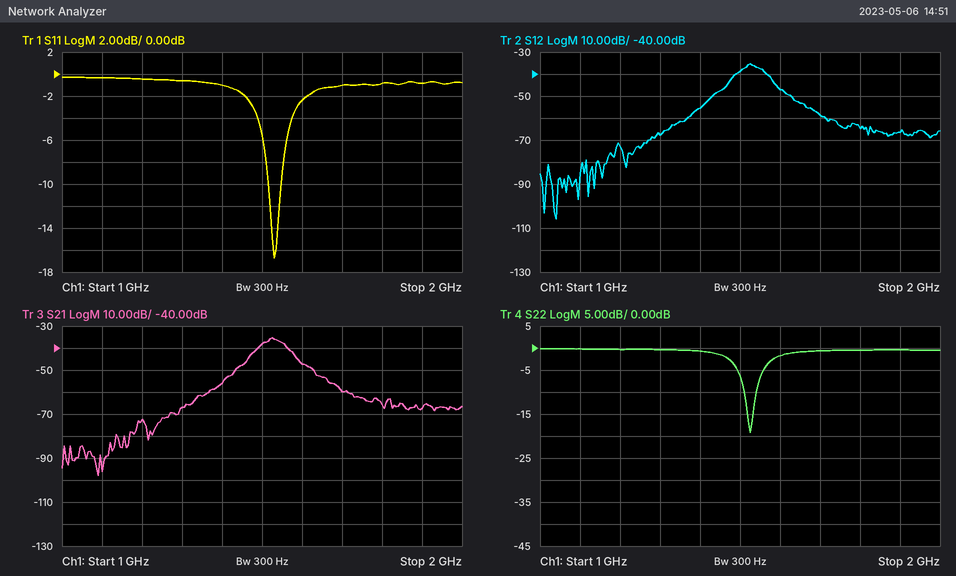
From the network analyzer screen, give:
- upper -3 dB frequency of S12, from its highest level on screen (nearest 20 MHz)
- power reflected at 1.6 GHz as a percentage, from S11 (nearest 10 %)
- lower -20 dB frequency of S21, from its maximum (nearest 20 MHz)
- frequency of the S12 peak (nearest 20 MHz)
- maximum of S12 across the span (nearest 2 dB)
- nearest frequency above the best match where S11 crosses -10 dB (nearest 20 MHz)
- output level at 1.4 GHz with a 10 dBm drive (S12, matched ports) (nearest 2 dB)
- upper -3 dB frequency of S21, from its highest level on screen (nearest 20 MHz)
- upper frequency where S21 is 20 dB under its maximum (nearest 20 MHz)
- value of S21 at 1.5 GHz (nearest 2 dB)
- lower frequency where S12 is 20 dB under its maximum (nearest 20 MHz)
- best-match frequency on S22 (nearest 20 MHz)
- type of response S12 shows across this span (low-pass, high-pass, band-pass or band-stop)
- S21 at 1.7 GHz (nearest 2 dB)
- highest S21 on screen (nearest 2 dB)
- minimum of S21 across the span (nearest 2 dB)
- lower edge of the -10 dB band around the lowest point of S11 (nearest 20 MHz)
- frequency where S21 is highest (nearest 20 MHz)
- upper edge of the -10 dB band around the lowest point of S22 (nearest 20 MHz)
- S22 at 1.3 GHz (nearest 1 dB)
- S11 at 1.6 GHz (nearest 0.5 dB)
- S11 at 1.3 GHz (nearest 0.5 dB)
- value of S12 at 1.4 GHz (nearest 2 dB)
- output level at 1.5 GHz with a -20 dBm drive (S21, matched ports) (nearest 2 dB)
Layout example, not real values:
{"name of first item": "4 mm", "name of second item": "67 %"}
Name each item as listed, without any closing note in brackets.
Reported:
{"upper -3 dB frequency of S12, from its highest level on screen": "1.56 GHz", "power reflected at 1.6 GHz as a percentage, from S11": "60 %", "lower -20 dB frequency of S21, from its maximum": "1.40 GHz", "frequency of the S12 peak": "1.52 GHz", "maximum of S12 across the span": "-36 dB", "nearest frequency above the best match where S11 crosses -10 dB": "1.54 GHz", "output level at 1.4 GHz with a 10 dBm drive (S12, matched ports)": "-46 dBm", "upper -3 dB frequency of S21, from its highest level on screen": "1.56 GHz", "upper frequency where S21 is 20 dB under its maximum": "1.66 GHz", "value of S21 at 1.5 GHz": "-38 dB", "lower frequency where S12 is 20 dB under its maximum": "1.40 GHz", "best-match frequency on S22": "1.52 GHz", "type of response S12 shows across this span": "band-pass", "S21 at 1.7 GHz": "-60 dB", "highest S21 on screen": "-36 dB", "minimum of S21 across the span": "-98 dB", "lower edge of the -10 dB band around the lowest point of S11": "1.52 GHz", "frequency where S21 is highest": "1.52 GHz", "upper edge of the -10 dB band around the lowest point of S22": "1.54 GHz", "S22 at 1.3 GHz": "0 dB", "S11 at 1.6 GHz": "-2.5 dB", "S11 at 1.3 GHz": "-0.5 dB", "value of S12 at 1.4 GHz": "-56 dB", "output level at 1.5 GHz with a -20 dBm drive (S21, matched ports)": "-58 dBm"}
